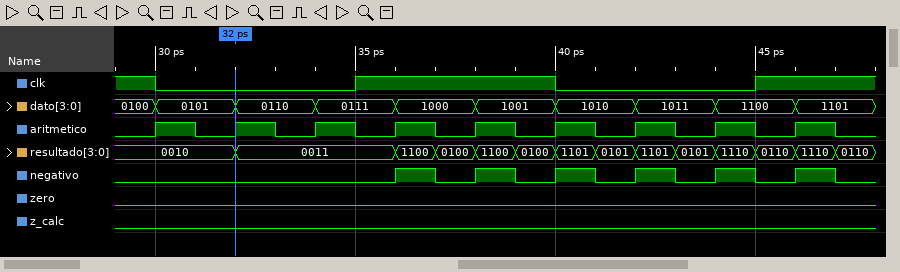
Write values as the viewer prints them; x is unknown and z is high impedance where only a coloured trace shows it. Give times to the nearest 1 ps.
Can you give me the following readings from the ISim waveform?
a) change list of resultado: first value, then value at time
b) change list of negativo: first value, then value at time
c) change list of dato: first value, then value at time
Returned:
0010, 0011 at 32 ps, 1100 at 36 ps, 0100 at 37 ps, 1100 at 38 ps, 0100 at 39 ps, 1101 at 40 ps, 0101 at 41 ps, 1101 at 42 ps, 0101 at 43 ps, 1110 at 44 ps, 0110 at 45 ps, 1110 at 46 ps, 0110 at 47 ps
0, 1 at 36 ps, 0 at 37 ps, 1 at 38 ps, 0 at 39 ps, 1 at 40 ps, 0 at 41 ps, 1 at 42 ps, 0 at 43 ps, 1 at 44 ps, 0 at 45 ps, 1 at 46 ps, 0 at 47 ps
0100, 0101 at 30 ps, 0110 at 32 ps, 0111 at 34 ps, 1000 at 36 ps, 1001 at 38 ps, 1010 at 40 ps, 1011 at 42 ps, 1100 at 44 ps, 1101 at 46 ps
